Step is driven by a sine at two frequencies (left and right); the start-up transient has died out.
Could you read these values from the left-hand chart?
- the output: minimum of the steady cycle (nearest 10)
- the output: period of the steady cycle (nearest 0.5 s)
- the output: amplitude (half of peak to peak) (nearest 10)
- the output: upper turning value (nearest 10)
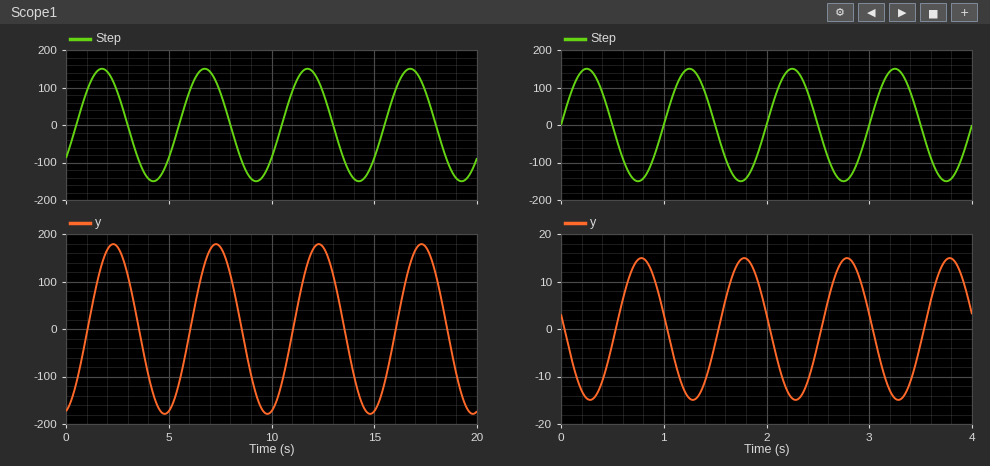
-180
5.0 s
180
180
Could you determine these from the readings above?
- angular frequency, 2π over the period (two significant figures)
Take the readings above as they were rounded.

1.3 rad/s
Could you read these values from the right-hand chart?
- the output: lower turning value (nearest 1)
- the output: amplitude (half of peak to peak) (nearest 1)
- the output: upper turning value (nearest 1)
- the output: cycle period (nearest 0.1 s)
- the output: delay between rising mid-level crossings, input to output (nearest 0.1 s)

-15
15
15
1.0 s
0.5 s
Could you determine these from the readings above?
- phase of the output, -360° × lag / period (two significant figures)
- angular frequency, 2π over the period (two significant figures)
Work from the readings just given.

-180°
6.3 rad/s
